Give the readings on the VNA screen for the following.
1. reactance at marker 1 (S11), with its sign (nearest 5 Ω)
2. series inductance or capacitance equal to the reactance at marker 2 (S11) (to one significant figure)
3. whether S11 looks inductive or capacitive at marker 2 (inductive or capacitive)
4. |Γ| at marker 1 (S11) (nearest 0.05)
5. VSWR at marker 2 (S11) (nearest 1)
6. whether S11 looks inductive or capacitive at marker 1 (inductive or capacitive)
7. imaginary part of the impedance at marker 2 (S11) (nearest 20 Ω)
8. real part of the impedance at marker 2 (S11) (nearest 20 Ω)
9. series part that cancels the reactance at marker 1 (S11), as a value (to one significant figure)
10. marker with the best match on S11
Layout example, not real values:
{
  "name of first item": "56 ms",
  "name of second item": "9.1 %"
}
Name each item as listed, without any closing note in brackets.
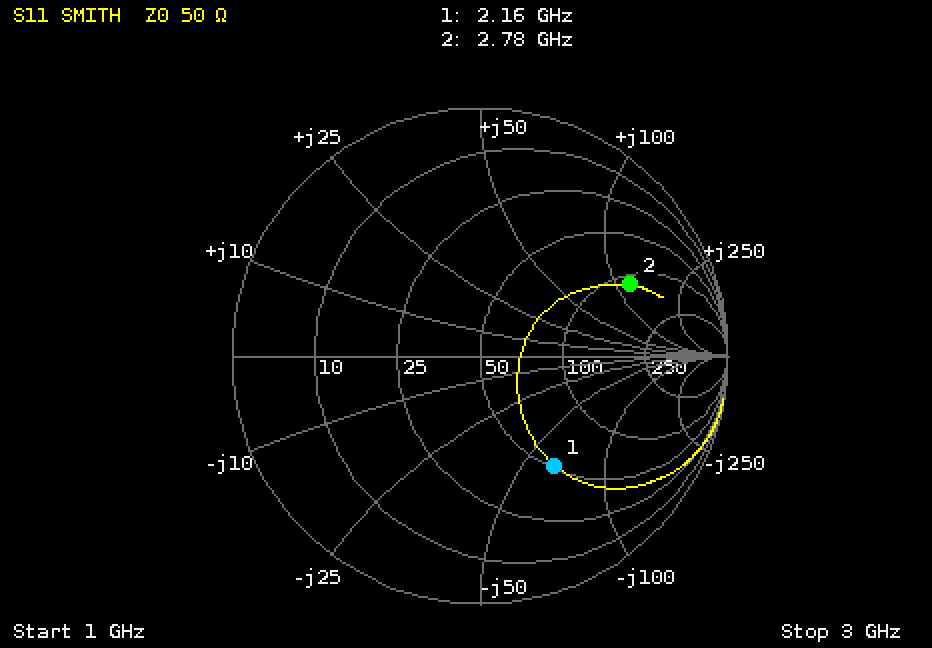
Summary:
{
  "reactance at marker 1 (S11), with its sign": "-65 Ω",
  "series inductance or capacitance equal to the reactance at marker 2 (S11)": "7 nH",
  "whether S11 looks inductive or capacitive at marker 2": "inductive",
  "|Γ| at marker 1 (S11)": "0.55",
  "VSWR at marker 2 (S11)": "5",
  "whether S11 looks inductive or capacitive at marker 1": "capacitive",
  "imaginary part of the impedance at marker 2 (S11)": "+120 Ω",
  "real part of the impedance at marker 2 (S11)": "120 Ω",
  "series part that cancels the reactance at marker 1 (S11), as a value": "5 nH",
  "marker with the best match on S11": "marker 1"
}
